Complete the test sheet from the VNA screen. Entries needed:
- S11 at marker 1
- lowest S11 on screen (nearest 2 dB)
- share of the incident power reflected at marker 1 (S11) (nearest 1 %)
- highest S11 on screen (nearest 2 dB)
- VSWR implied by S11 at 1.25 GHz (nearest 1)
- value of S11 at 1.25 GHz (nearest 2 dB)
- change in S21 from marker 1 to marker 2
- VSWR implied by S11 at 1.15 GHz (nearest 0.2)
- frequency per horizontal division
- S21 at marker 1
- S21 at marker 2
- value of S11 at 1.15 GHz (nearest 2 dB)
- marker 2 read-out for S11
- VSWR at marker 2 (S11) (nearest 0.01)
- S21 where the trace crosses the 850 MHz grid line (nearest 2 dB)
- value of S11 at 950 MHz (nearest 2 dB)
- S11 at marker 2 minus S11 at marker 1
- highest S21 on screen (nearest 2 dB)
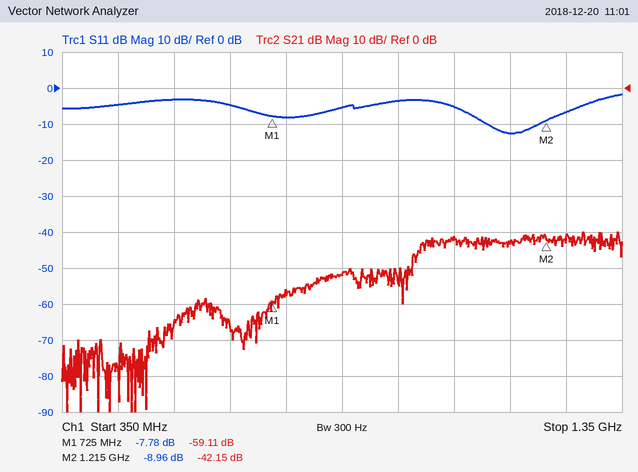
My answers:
-7.78 dB
-12 dB
17 %
-2 dB
3
-6 dB
16.96 dB
1.6
100 MHz
-59.11 dB
-42.15 dB
-12 dB
-8.96 dB
2.11
-52 dB
-4 dB
-1.18 dB
-40 dB
